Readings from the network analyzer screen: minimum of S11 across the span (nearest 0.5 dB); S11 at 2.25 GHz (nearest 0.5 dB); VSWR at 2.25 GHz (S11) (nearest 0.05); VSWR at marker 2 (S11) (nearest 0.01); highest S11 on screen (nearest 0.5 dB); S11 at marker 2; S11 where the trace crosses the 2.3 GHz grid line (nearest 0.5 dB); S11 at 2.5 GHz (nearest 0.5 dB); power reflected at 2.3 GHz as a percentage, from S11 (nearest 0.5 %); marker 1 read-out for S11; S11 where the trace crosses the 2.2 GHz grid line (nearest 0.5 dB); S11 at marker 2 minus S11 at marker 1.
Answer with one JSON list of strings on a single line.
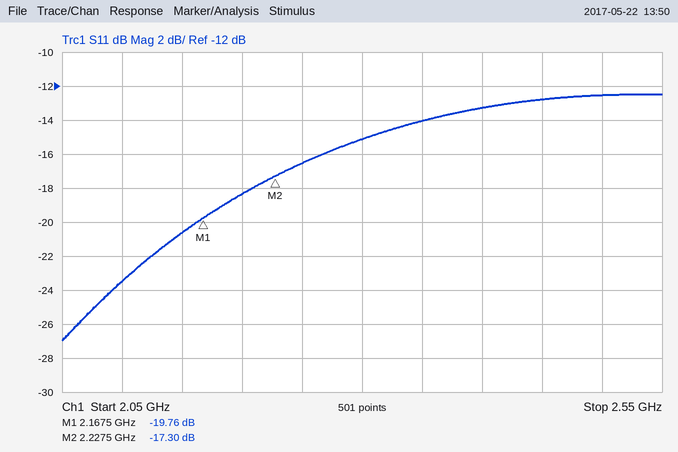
["-27.0 dB", "-16.5 dB", "1.35", "1.32", "-12.5 dB", "-17.30 dB", "-15.0 dB", "-12.5 dB", "3.0 %", "-19.76 dB", "-18.5 dB", "2.46 dB"]
